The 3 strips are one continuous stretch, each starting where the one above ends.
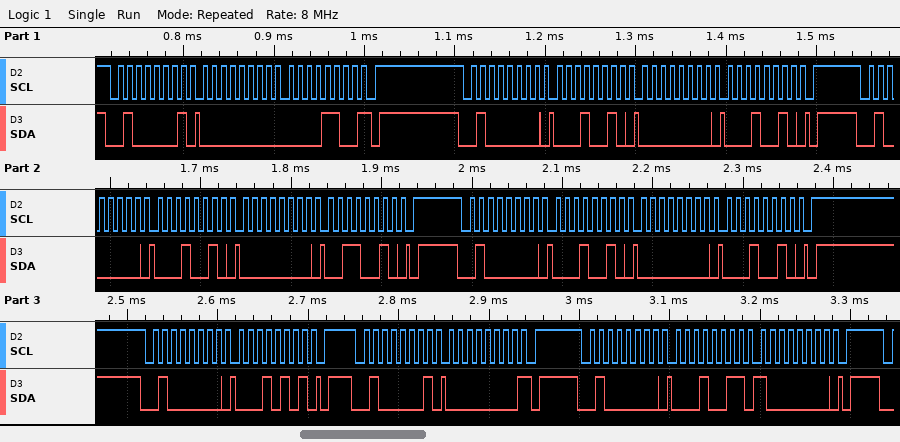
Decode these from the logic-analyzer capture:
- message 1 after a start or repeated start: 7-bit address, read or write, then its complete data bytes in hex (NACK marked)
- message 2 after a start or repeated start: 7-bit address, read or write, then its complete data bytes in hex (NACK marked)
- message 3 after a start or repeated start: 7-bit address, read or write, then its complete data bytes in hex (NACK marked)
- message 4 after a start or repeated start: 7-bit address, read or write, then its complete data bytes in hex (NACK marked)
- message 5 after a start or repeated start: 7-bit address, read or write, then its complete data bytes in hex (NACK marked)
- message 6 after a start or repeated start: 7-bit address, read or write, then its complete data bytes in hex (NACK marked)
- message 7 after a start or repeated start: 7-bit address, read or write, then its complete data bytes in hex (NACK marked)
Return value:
0x20 read: 00 0C NACK
0x20 write: 12 00 12
0x20 write: 12 00 32
0x20 write: 12 00 12
0x20 write: 15
0x20 read: 00 NACK
0x20 write: 13 80
